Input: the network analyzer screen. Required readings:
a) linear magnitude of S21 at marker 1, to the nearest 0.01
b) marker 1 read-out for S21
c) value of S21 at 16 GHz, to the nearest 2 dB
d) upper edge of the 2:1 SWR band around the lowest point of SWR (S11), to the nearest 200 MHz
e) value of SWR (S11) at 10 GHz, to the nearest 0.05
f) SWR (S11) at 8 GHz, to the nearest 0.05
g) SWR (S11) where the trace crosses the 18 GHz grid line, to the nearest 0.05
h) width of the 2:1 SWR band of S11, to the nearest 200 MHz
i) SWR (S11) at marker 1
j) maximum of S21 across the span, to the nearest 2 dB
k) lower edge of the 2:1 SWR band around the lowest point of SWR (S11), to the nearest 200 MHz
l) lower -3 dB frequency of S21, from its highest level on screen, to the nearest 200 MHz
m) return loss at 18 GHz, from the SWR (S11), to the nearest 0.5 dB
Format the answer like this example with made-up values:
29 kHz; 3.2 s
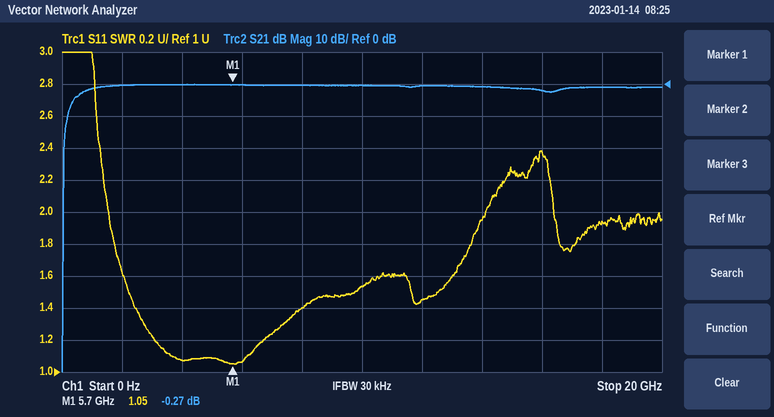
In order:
0.97; -0.27 dB; -2 dB; 14.2 GHz; 1.55; 1.40; 1.95; 12.6 GHz; 1.05; 0 dB; 1.6 GHz; 600 MHz; 10.0 dB
